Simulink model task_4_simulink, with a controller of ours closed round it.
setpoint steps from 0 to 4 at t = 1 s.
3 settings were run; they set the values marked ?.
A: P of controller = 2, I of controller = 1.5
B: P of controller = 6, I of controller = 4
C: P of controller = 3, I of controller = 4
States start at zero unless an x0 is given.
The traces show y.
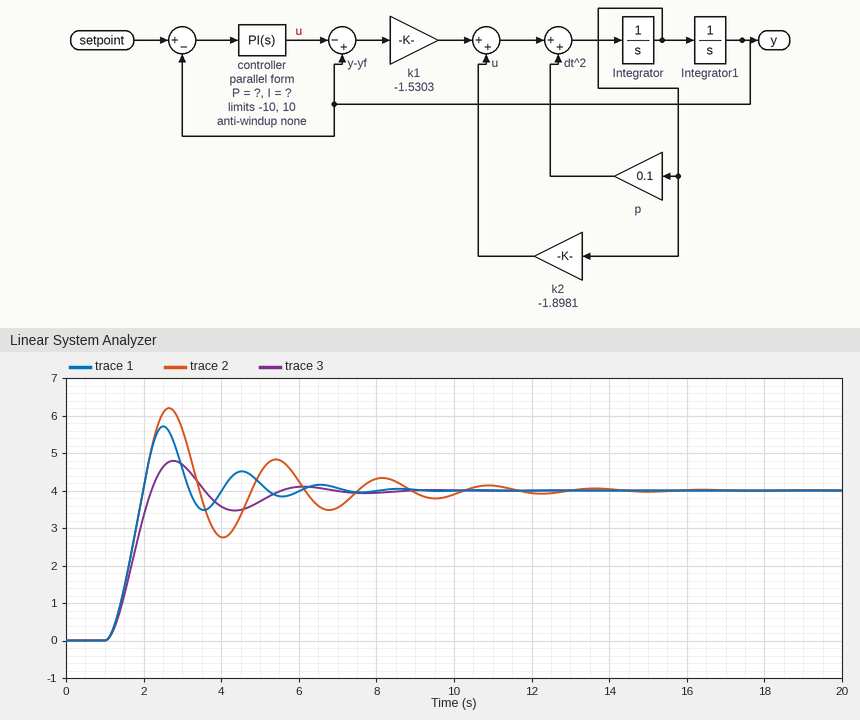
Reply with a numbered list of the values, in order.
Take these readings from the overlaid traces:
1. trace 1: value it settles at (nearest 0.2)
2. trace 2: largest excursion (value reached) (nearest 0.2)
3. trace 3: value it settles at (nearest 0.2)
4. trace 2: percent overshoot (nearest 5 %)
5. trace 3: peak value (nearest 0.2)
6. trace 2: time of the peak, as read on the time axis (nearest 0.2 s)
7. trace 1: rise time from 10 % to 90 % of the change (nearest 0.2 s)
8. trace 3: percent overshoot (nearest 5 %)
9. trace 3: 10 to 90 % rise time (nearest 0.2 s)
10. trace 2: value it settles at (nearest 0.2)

1. 4.0
2. 6.2
3. 4.0
4. 55 %
5. 4.8
6. 2.6 s
7. 0.6 s
8. 20 %
9. 0.8 s
10. 4.0
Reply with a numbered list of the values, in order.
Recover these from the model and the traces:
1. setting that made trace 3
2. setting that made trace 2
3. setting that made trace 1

1. A
2. C
3. B
